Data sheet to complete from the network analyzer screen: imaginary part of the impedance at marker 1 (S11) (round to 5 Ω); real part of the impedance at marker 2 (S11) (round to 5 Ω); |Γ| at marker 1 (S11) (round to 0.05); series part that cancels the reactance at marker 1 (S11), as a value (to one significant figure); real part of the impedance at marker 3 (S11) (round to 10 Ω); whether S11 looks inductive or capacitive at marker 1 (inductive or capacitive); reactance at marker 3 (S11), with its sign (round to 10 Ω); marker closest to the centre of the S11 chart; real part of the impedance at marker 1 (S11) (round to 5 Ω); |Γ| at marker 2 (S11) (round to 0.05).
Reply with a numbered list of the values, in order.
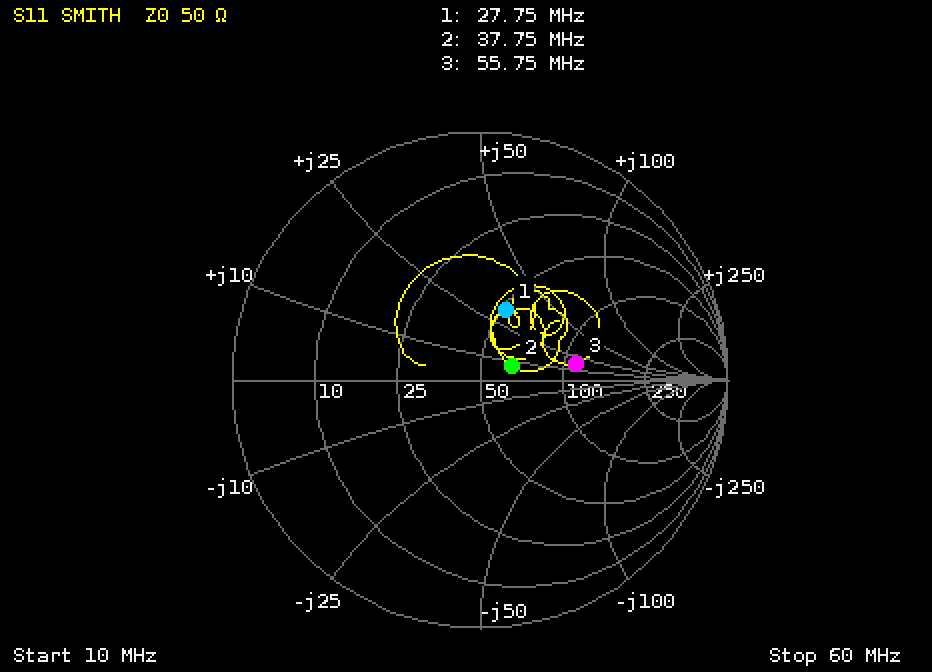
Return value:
1. +30 Ω
2. 65 Ω
3. 0.30
4. 200 pF
5. 110 Ω
6. inductive
7. +20 Ω
8. marker 2
9. 50 Ω
10. 0.15
